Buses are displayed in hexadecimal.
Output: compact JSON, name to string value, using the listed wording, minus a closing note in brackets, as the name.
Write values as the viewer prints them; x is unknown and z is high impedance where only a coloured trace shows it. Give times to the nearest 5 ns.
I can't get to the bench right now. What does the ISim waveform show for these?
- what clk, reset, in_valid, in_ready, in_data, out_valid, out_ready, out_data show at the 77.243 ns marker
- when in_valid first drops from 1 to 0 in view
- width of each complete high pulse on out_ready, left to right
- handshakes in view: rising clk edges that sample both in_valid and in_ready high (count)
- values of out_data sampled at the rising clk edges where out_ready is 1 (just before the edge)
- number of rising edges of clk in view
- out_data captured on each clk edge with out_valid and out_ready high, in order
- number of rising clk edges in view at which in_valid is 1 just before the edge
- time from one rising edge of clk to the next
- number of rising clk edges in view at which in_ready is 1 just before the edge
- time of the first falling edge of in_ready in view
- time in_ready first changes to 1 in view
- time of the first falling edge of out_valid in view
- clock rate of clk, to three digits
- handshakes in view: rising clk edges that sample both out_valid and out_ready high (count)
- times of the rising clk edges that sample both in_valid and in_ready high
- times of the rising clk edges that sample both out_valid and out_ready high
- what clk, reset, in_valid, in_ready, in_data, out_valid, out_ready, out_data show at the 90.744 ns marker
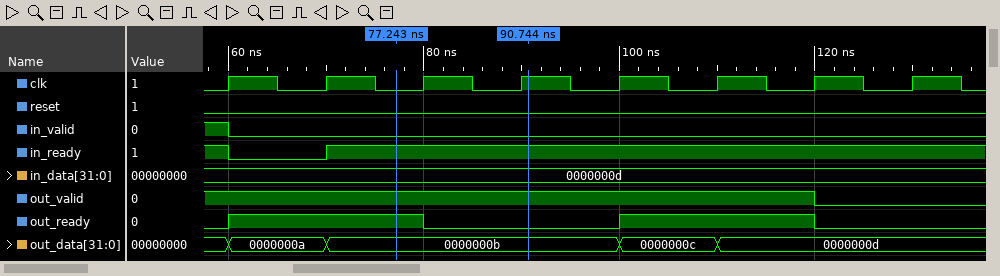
{"what clk, reset, in_valid, in_ready, in_data, out_valid, out_ready, out_data show at the 77.243 ns marker": "clk=0, reset=0, in_valid=0, in_ready=1, in_data=0000000d, out_valid=1, out_ready=1, out_data=0000000b", "when in_valid first drops from 1 to 0 in view": "60 ns", "width of each complete high pulse on out_ready, left to right": "20 ns, 20 ns", "handshakes in view: rising clk edges that sample both in_valid and in_ready high": "1", "values of out_data sampled at the rising clk edges where out_ready is 1": "0000000a, 0000000b, 0000000c, 0000000d", "number of rising edges of clk in view": "8", "out_data captured on each clk edge with out_valid and out_ready high, in order": "0000000a, 0000000b, 0000000c, 0000000d", "number of rising clk edges in view at which in_valid is 1 just before the edge": "1", "time from one rising edge of clk to the next": "10 ns", "number of rising clk edges in view at which in_ready is 1 just before the edge": "7", "time of the first falling edge of in_ready in view": "60 ns", "time in_ready first changes to 1 in view": "70 ns", "time of the first falling edge of out_valid in view": "120 ns", "clock rate of clk, to three digits": "100 MHz", "handshakes in view: rising clk edges that sample both out_valid and out_ready high": "4", "times of the rising clk edges that sample both in_valid and in_ready high": "60 ns", "times of the rising clk edges that sample both out_valid and out_ready high": "70 ns, 80 ns, 110 ns, 120 ns", "what clk, reset, in_valid, in_ready, in_data, out_valid, out_ready, out_data show at the 90.744 ns marker": "clk=1, reset=0, in_valid=0, in_ready=1, in_data=0000000d, out_valid=1, out_ready=0, out_data=0000000b"}
